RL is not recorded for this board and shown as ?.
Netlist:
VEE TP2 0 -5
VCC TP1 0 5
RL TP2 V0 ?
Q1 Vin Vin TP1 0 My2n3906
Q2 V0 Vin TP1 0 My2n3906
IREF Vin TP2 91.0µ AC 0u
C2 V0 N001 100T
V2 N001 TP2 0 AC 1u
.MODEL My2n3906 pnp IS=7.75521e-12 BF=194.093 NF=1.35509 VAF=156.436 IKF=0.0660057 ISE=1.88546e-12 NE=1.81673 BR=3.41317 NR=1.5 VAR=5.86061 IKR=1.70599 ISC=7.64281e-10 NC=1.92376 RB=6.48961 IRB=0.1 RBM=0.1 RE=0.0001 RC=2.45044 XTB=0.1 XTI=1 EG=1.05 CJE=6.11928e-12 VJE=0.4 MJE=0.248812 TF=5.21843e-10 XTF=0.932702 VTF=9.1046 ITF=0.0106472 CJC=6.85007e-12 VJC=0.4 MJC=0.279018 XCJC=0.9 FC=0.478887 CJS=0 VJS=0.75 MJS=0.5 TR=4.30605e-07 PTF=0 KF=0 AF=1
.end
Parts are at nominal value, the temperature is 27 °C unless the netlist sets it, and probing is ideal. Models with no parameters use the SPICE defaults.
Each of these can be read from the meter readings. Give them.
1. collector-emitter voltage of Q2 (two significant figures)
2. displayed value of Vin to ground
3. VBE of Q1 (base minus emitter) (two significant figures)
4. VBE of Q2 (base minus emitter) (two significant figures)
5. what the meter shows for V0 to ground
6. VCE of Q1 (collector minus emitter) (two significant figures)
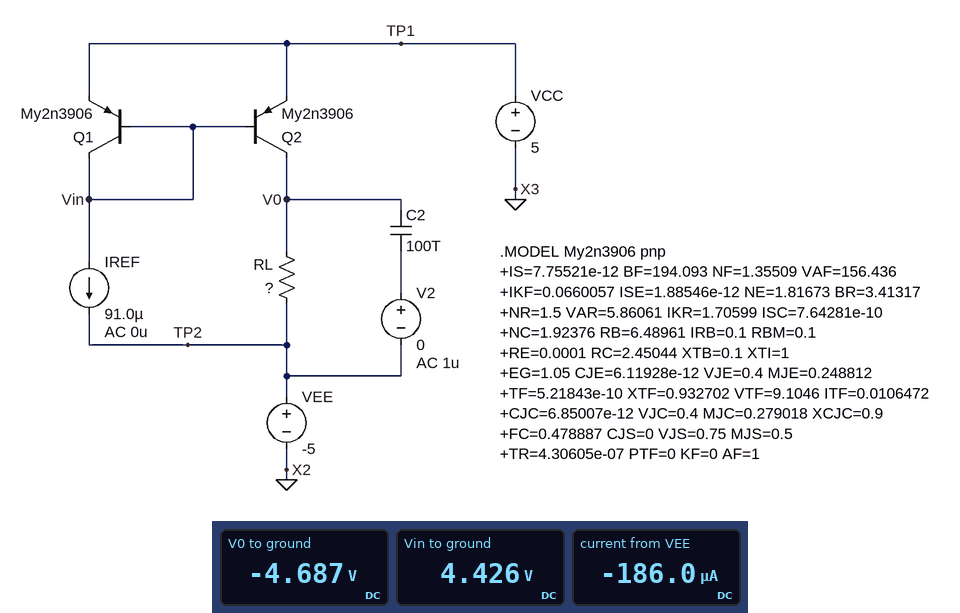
-9.7 V
4.426 V
-570 mV
-570 mV
-4.687 V
-570 mV
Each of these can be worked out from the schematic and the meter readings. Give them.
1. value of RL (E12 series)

3.3 kΩ
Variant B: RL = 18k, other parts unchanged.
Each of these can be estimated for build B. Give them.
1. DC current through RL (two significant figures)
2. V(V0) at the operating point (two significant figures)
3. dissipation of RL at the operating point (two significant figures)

94 µA
-3.3 V
160 µW
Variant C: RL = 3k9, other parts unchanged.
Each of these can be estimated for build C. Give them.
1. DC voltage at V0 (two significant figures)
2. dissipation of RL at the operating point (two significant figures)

-4.6 V
35 µW
